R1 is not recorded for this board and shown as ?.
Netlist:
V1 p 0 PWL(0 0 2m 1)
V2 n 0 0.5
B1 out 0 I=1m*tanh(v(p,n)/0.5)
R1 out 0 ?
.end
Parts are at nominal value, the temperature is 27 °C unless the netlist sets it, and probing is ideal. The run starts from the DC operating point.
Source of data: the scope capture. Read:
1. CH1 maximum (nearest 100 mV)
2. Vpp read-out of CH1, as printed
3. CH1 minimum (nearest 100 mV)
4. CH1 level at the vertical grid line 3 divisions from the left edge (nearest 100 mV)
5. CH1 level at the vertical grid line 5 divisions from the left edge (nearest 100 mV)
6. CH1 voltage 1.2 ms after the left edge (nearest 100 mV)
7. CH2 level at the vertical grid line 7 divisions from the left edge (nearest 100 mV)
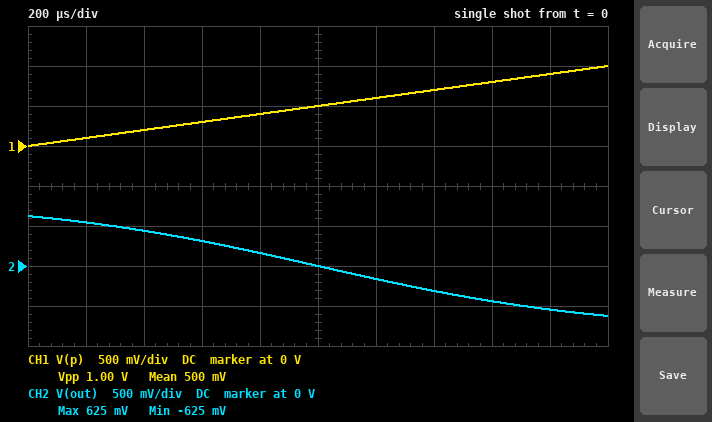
1.0 V
1.00 V
0 V
300 mV
500 mV
600 mV
-300 mV
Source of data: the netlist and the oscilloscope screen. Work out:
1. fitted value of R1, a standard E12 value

820 Ω
